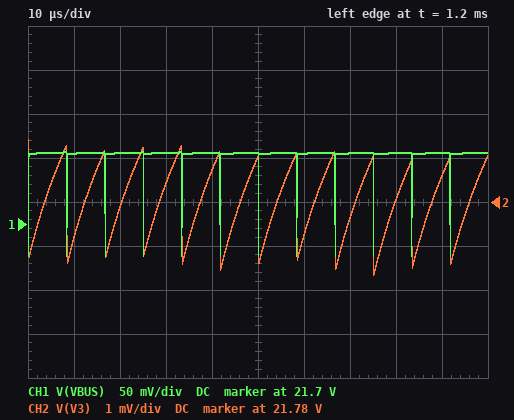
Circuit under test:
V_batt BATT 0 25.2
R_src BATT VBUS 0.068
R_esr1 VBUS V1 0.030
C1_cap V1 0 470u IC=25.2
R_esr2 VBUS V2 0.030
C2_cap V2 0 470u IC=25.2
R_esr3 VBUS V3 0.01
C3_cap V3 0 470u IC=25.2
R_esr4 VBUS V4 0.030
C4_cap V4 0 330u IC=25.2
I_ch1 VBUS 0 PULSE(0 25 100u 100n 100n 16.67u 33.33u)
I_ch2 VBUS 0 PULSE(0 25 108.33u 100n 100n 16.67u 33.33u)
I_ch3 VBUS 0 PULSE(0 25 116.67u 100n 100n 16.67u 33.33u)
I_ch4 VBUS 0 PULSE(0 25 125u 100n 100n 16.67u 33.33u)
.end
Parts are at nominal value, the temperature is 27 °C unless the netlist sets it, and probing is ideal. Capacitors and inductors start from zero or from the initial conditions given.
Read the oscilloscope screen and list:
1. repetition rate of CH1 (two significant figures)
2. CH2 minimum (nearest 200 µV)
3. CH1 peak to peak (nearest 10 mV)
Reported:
120 kHz
21.7774 V
120 mV
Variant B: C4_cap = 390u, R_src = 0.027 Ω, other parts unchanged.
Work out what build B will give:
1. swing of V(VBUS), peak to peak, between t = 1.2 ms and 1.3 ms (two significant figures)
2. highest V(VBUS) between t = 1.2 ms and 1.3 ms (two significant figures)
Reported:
110 mV
24 V
